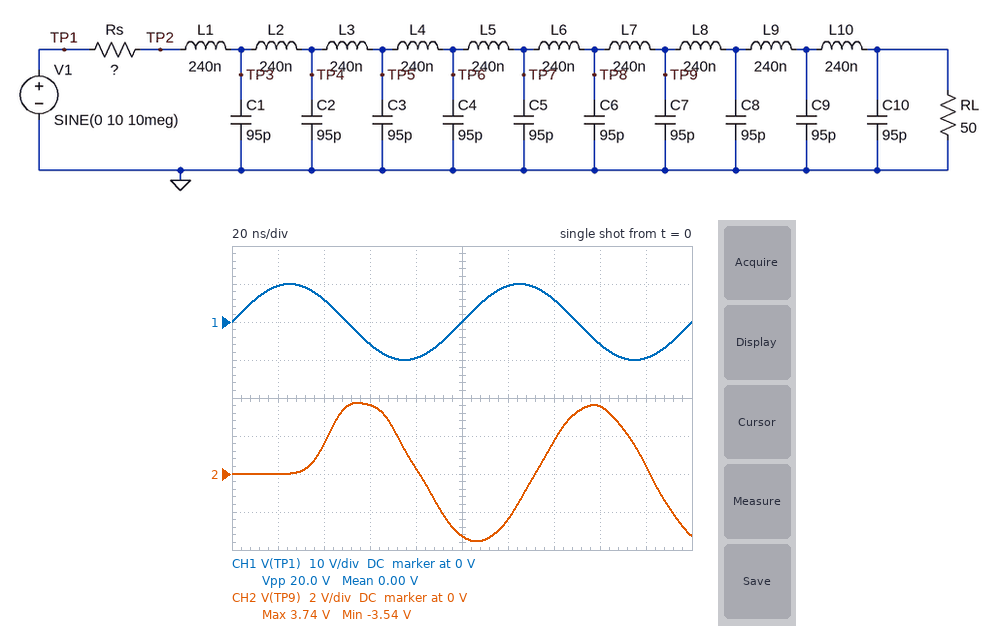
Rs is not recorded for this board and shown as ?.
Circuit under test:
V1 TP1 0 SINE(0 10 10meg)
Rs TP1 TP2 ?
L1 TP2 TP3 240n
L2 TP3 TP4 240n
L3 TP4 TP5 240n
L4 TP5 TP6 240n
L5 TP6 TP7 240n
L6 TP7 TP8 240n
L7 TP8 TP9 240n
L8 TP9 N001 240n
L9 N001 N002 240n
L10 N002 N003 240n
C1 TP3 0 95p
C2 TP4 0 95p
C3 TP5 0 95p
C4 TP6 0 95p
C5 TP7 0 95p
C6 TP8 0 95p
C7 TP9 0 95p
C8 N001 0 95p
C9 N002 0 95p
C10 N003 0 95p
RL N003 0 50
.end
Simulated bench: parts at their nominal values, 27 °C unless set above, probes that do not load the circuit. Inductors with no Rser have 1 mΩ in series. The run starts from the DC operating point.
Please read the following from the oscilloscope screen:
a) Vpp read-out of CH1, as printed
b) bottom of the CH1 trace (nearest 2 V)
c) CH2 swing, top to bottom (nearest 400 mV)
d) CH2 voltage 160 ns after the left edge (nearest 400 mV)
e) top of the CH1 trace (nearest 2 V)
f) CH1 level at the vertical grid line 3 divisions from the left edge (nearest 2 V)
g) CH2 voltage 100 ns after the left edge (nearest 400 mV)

20.0 V
-10 V
7.2 V
3.6 V
10 V
-6 V
-3.2 V
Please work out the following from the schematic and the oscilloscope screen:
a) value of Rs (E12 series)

82 Ω
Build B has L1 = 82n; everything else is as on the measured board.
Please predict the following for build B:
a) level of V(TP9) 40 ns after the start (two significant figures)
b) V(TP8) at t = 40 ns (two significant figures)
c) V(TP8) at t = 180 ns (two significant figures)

1.9 V
3.0 V
-1.1 V
